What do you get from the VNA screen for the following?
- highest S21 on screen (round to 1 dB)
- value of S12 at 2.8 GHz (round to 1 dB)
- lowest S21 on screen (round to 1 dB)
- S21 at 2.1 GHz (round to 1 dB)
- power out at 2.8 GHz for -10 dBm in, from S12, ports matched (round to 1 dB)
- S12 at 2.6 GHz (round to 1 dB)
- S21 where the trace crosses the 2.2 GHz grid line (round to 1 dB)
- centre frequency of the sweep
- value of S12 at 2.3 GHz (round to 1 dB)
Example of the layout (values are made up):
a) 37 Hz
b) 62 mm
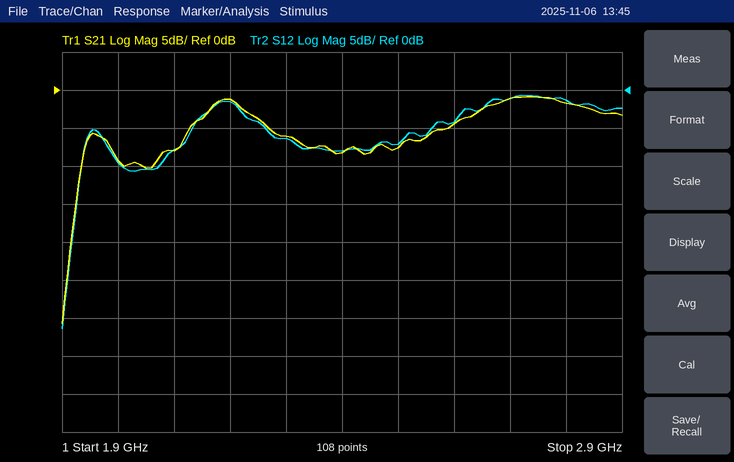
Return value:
a) -1 dB
b) -1 dB
c) -31 dB
d) -8 dB
e) -11 dBm
f) -4 dB
g) -1 dB
h) 2.4 GHz
i) -6 dB
